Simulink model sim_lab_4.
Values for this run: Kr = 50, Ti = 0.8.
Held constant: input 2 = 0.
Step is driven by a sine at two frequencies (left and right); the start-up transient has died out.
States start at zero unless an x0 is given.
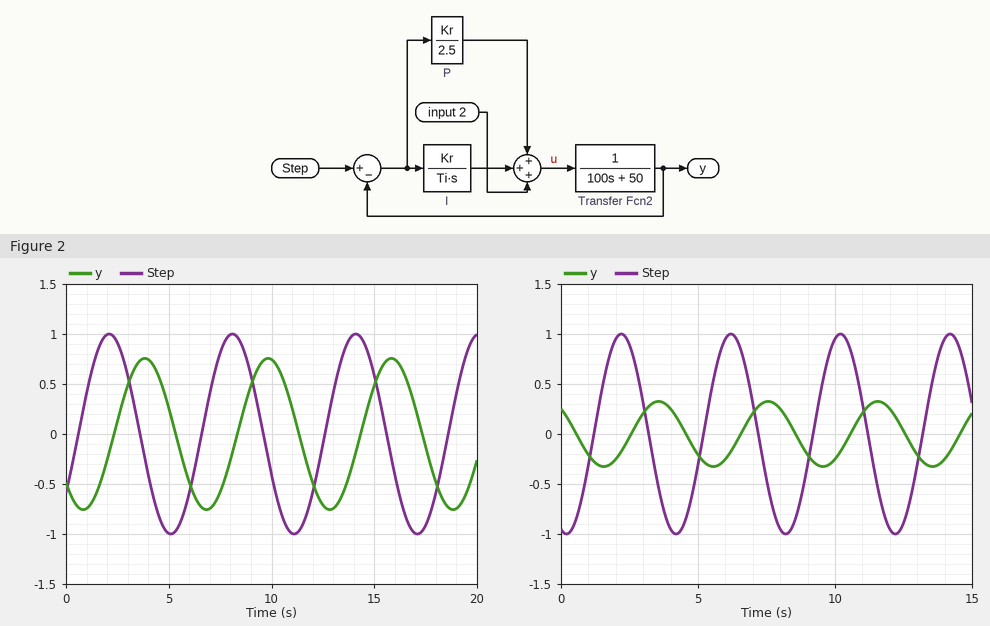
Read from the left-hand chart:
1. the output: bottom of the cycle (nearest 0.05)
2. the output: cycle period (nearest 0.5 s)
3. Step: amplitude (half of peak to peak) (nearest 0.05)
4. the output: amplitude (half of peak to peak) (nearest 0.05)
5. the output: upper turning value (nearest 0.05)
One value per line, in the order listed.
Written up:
-0.75
6.0 s
1.00
0.75
0.75
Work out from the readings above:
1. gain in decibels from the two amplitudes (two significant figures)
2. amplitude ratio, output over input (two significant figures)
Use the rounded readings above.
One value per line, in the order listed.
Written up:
-2.5 dB
0.75
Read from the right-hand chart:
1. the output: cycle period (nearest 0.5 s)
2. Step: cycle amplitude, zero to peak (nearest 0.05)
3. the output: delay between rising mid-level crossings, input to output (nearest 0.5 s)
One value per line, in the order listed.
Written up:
4.0 s
1.00
1.5 s
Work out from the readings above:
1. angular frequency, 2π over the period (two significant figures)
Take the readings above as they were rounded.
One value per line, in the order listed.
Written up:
1.6 rad/s
